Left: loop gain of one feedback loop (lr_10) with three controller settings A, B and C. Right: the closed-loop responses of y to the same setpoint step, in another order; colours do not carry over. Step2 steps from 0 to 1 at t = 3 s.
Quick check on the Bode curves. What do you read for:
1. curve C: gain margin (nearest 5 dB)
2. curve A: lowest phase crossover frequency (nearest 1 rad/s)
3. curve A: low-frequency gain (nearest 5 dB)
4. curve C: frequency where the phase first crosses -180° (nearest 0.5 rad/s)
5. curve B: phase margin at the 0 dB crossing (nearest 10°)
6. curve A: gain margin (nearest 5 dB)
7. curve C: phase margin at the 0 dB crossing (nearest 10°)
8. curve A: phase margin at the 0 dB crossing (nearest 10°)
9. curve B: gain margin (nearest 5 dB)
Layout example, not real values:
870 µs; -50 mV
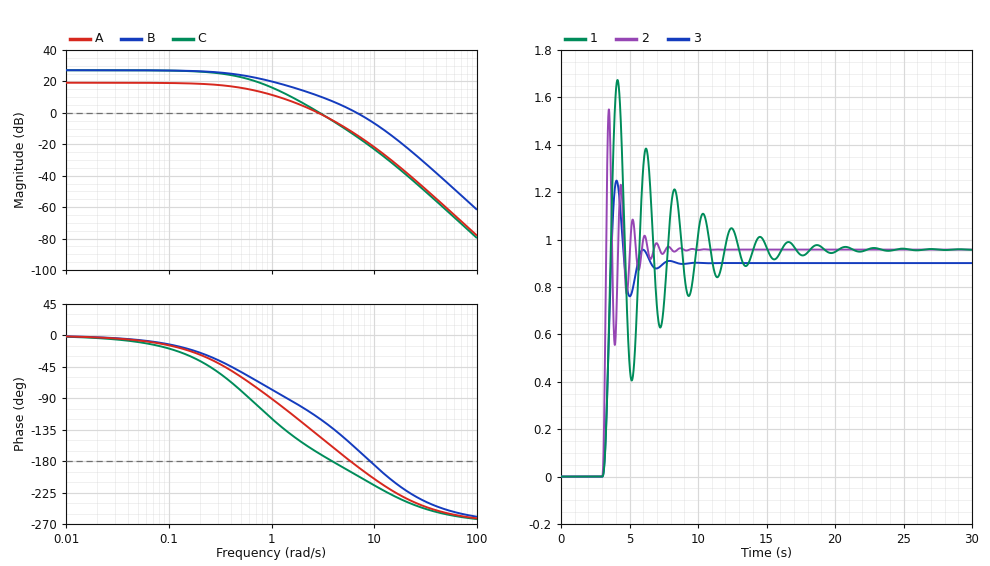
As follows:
5 dB; 6 rad/s; 20 dB; 4.0 rad/s; 20°; 10 dB; 10°; 40°; 5 dB
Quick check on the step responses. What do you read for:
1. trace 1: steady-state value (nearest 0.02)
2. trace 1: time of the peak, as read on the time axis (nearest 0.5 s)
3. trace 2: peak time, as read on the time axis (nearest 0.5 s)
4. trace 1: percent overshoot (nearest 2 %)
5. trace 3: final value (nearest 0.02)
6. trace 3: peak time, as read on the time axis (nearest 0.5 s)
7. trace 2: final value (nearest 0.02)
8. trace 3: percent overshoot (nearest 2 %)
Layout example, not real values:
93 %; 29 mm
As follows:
0.96; 4.0 s; 3.5 s; 74 %; 0.90; 4.0 s; 0.96; 38 %
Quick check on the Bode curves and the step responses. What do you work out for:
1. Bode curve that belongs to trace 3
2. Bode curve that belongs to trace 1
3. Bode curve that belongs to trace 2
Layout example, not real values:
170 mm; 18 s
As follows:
A; C; B
